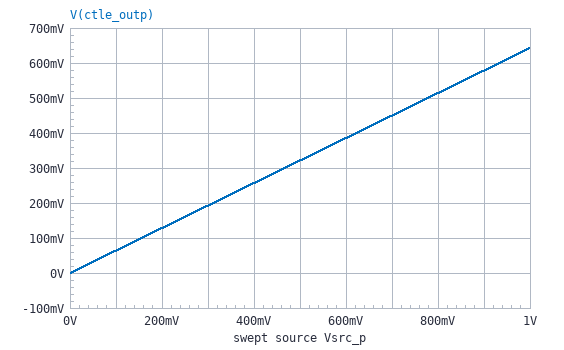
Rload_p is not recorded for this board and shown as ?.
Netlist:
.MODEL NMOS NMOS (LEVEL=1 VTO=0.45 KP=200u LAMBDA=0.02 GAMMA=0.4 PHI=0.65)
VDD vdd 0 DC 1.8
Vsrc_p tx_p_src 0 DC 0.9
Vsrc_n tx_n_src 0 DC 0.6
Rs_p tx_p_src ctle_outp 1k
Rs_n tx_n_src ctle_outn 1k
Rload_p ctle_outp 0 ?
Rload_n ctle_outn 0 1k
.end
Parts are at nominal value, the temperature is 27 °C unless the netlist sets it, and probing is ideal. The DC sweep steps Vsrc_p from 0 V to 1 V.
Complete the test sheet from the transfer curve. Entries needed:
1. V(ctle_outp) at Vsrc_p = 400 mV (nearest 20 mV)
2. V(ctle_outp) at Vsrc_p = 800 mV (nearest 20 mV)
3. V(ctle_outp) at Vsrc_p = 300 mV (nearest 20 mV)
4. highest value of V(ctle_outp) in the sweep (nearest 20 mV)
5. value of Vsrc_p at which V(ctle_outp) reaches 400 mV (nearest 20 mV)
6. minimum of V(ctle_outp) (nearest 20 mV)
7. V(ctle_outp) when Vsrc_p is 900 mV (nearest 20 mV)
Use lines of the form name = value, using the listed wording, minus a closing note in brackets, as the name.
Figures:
V(ctle_outp) at Vsrc_p = 400 mV = 260 mV
V(ctle_outp) at Vsrc_p = 800 mV = 520 mV
V(ctle_outp) at Vsrc_p = 300 mV = 200 mV
highest value of V(ctle_outp) in the sweep = 640 mV
value of Vsrc_p at which V(ctle_outp) reaches 400 mV = 620 mV
minimum of V(ctle_outp) = 0 V
V(ctle_outp) when Vsrc_p is 900 mV = 580 mV
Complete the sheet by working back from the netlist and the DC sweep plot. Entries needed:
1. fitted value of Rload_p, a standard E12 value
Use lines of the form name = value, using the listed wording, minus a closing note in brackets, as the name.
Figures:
fitted value of Rload_p, a standard E12 value = 1.8 kΩ
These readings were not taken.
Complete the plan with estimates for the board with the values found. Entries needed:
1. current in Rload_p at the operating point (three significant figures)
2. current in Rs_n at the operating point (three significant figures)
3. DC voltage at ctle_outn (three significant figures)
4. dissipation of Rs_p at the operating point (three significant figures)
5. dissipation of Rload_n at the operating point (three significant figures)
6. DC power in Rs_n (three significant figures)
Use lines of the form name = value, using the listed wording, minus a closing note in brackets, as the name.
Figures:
current in Rload_p at the operating point = 321 µA
current in Rs_n at the operating point = 300 µA
DC voltage at ctle_outn = 300 mV
dissipation of Rs_p at the operating point = 103 µW
dissipation of Rload_n at the operating point = 90.0 µW
DC power in Rs_n = 90.0 µW
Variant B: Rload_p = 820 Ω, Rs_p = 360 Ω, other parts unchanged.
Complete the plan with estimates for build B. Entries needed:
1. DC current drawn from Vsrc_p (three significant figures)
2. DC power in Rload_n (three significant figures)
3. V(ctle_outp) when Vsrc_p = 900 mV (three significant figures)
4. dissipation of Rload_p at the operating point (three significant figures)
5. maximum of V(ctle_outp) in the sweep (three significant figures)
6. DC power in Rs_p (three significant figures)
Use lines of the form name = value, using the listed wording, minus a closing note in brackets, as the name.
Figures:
DC current drawn from Vsrc_p = 763 µA
DC power in Rload_n = 90.0 µW
V(ctle_outp) when Vsrc_p = 900 mV = 625 mV
dissipation of Rload_p at the operating point = 477 µW
maximum of V(ctle_outp) in the sweep = 695 mV
DC power in Rs_p = 209 µW
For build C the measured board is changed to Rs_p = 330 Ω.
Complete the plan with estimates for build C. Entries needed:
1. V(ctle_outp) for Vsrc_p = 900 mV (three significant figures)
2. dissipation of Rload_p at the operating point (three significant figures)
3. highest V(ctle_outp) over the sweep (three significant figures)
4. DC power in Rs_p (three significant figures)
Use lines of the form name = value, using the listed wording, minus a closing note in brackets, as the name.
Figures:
V(ctle_outp) for Vsrc_p = 900 mV = 761 mV
dissipation of Rload_p at the operating point = 321 µW
highest V(ctle_outp) over the sweep = 845 mV
DC power in Rs_p = 58.9 µW
